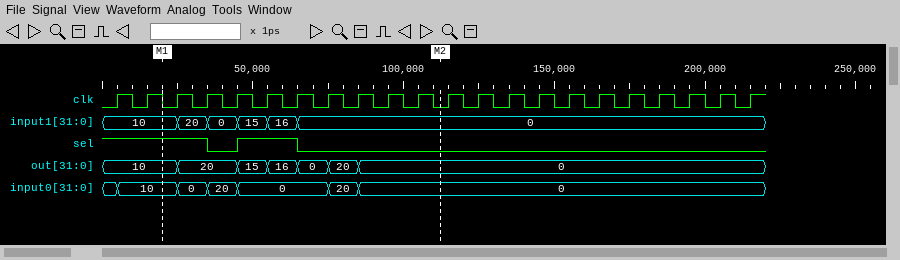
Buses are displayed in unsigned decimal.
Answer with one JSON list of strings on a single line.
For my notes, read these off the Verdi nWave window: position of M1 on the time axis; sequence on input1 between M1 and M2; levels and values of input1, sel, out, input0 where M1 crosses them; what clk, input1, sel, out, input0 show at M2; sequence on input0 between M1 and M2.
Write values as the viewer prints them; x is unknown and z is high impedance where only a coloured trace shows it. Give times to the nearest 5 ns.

["20 ns", "10, 20, 0, 15, 16, 0", "input1=10, sel=1, out=10, input0=10", "clk=0, input1=0, sel=0, out=0, input0=0", "10, 0, 20, 0, 20, 0"]
